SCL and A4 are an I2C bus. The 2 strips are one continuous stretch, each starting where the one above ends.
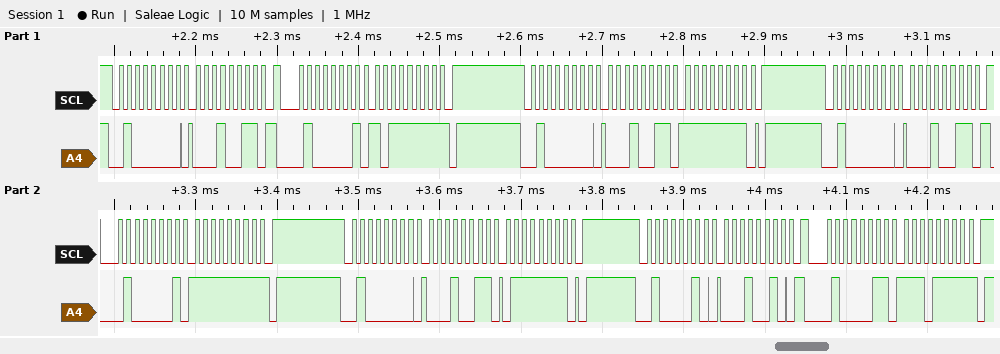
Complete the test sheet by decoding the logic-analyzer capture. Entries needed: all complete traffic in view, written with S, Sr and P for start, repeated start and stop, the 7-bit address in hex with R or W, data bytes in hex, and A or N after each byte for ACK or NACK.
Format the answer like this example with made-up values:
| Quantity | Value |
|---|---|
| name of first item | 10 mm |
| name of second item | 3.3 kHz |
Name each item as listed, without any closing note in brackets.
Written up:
| Quantity | Value |
|---|---|
| all complete traffic in view, written with S, Sr and P for start, repeated start and stop, the 7-bit address in hex with R or W, data bytes in hex, and A or N after each byte for ACK or NACK | S 20W A 13 A Sr 20R A BF N P S 20W A 13 A FF A P S 20W A 13 A Sr 20R A FF N P S 20W A 13 A 7F A P S 21W A 12 A Sr 21R A EF N P |
